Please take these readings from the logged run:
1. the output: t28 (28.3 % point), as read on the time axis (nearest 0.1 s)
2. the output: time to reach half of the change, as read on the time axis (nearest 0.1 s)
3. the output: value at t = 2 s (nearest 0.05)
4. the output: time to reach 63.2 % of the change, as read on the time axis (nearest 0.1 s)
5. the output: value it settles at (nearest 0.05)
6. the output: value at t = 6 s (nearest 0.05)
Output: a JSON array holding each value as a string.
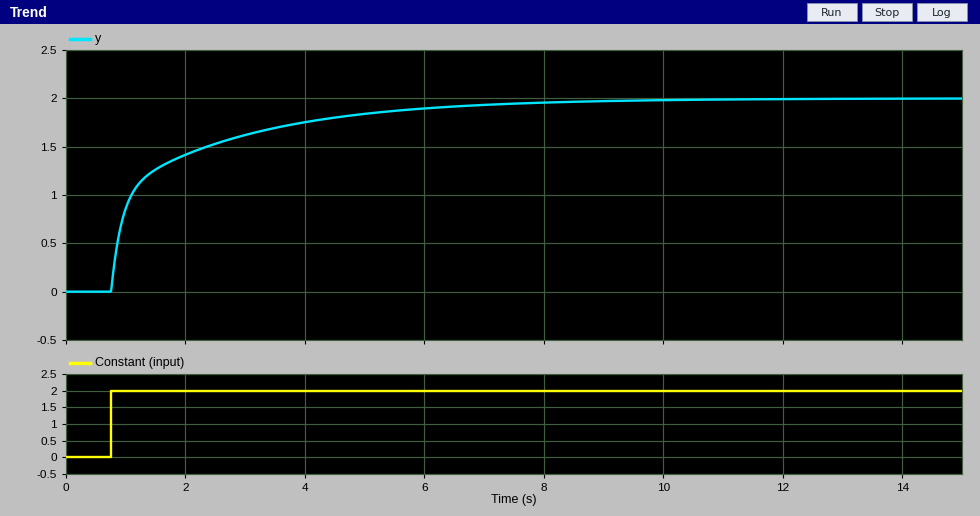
["0.9 s", "1.1 s", "1.40", "1.5 s", "2.00", "1.90"]
